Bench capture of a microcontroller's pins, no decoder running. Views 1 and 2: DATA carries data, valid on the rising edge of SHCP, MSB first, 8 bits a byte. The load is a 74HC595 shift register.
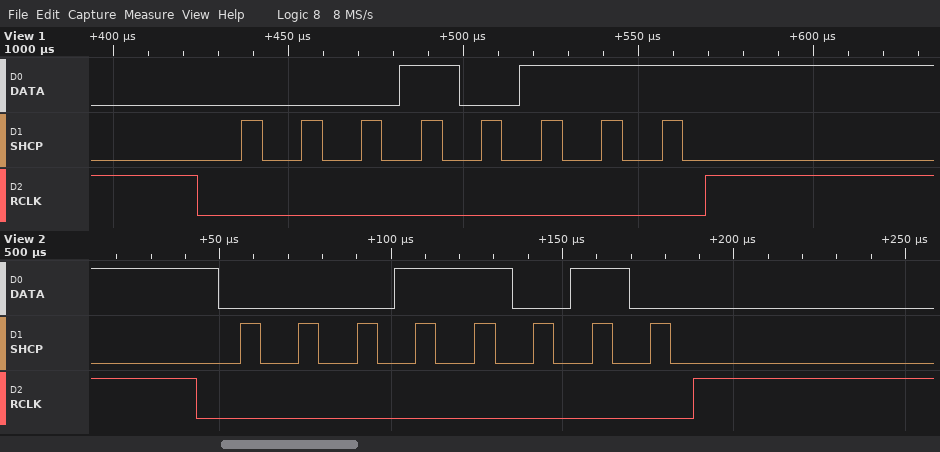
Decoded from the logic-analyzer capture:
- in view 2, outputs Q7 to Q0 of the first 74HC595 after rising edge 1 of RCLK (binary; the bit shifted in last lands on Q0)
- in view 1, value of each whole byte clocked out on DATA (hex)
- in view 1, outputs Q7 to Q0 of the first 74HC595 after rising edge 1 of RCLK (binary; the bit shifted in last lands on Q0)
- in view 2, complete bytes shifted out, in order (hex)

00011010
17
00010111
0x1A
